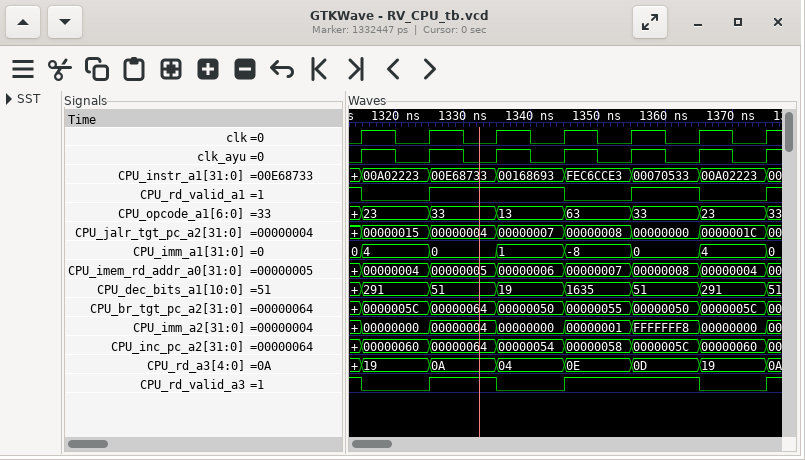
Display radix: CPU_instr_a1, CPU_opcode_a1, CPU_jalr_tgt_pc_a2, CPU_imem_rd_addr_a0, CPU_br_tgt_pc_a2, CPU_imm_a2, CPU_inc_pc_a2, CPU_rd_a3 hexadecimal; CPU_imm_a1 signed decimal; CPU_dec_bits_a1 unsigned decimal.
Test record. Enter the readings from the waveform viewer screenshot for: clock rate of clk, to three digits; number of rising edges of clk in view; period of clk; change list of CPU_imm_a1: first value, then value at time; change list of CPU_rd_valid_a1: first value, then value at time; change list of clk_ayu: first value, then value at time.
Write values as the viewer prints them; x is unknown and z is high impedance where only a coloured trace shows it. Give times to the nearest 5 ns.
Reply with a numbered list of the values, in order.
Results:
1. 100 MHz
2. 7
3. 10 ns
4. 0, 4 at 1315 ns, 0 at 1325 ns, 1 at 1335 ns, -8 at 1345 ns, 0 at 1355 ns, 4 at 1365 ns, 0 at 1375 ns
5. 1, 0 at 1315 ns, 1 at 1325 ns, 0 at 1345 ns, 1 at 1355 ns, 0 at 1365 ns, 1 at 1375 ns
6. 0, 1 at 1315 ns, 0 at 1320 ns, 1 at 1325 ns, 0 at 1330 ns, 1 at 1335 ns, 0 at 1340 ns, 1 at 1345 ns, 0 at 1350 ns, 1 at 1355 ns, 0 at 1360 ns, 1 at 1365 ns, 0 at 1370 ns, 1 at 1375 ns
